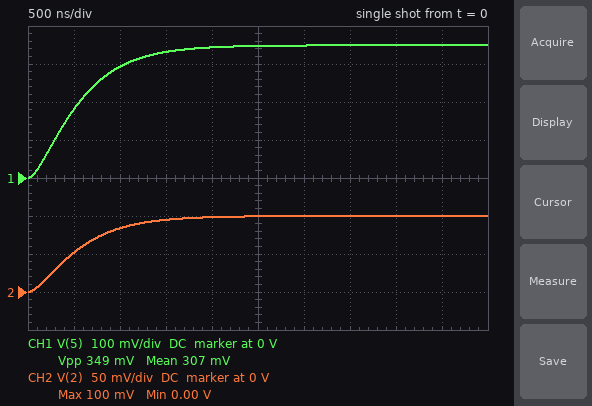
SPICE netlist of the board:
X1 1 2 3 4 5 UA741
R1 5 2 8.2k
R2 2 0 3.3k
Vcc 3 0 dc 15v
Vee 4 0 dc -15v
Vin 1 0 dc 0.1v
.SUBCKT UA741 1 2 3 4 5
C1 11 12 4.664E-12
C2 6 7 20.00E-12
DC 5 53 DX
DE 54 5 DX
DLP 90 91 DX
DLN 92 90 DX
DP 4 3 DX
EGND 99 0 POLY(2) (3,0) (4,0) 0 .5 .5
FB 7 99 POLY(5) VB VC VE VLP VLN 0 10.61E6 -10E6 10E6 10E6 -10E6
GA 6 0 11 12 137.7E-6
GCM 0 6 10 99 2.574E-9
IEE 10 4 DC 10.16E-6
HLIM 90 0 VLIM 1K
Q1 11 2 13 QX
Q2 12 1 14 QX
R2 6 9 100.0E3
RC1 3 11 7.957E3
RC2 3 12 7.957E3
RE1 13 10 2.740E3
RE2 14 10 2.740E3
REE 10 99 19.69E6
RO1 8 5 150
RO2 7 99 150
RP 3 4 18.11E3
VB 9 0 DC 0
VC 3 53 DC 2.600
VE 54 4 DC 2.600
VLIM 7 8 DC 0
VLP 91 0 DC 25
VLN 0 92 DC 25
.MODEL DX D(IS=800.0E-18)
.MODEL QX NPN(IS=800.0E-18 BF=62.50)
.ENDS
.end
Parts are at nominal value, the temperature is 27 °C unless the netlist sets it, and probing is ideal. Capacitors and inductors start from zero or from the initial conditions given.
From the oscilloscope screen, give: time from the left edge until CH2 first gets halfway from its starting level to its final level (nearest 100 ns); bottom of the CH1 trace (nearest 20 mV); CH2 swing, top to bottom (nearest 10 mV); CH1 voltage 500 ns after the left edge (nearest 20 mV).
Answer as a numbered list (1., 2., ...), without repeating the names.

1. 500 ns
2. 0 V
3. 100 mV
4. 180 mV
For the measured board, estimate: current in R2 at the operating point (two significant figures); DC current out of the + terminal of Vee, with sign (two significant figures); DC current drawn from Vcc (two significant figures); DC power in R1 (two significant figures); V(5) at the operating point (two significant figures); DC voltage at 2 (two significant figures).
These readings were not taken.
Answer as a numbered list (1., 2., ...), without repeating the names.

1. 30 µA
2. -1.7 mA
3. 1.7 mA
4. 7.6 µW
5. 350 mV
6. 100 mV
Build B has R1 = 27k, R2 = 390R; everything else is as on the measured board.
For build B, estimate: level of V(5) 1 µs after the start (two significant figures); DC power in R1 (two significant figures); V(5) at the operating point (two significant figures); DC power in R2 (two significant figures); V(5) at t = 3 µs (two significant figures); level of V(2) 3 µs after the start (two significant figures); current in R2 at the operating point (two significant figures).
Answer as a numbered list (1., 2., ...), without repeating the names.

1. 450 mV
2. 1.8 mW
3. 7.0 V
4. 26 µW
5. 1.4 V
6. 19 mV
7. 260 µA
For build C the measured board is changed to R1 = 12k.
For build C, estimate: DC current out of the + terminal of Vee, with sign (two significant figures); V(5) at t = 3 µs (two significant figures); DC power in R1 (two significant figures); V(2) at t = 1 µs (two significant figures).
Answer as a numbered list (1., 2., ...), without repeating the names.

1. -1.7 mA
2. 460 mV
3. 11 µW
4. 72 mV
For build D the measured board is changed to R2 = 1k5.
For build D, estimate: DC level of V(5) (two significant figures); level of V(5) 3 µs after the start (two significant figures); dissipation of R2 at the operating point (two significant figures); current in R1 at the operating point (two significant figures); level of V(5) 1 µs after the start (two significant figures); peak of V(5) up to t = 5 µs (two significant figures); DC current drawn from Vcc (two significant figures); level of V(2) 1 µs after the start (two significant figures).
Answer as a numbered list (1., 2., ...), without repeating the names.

1. 650 mV
2. 620 mV
3. 6.7 µW
4. 67 µA
5. 370 mV
6. 640 mV
7. 1.7 mA
8. 57 mV
